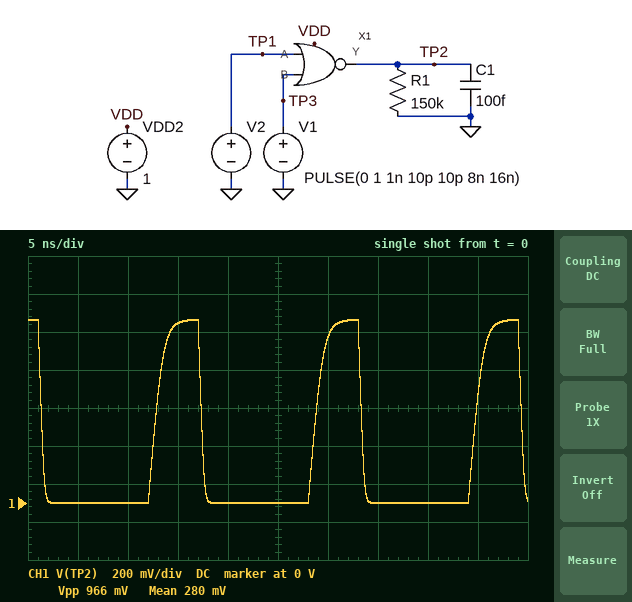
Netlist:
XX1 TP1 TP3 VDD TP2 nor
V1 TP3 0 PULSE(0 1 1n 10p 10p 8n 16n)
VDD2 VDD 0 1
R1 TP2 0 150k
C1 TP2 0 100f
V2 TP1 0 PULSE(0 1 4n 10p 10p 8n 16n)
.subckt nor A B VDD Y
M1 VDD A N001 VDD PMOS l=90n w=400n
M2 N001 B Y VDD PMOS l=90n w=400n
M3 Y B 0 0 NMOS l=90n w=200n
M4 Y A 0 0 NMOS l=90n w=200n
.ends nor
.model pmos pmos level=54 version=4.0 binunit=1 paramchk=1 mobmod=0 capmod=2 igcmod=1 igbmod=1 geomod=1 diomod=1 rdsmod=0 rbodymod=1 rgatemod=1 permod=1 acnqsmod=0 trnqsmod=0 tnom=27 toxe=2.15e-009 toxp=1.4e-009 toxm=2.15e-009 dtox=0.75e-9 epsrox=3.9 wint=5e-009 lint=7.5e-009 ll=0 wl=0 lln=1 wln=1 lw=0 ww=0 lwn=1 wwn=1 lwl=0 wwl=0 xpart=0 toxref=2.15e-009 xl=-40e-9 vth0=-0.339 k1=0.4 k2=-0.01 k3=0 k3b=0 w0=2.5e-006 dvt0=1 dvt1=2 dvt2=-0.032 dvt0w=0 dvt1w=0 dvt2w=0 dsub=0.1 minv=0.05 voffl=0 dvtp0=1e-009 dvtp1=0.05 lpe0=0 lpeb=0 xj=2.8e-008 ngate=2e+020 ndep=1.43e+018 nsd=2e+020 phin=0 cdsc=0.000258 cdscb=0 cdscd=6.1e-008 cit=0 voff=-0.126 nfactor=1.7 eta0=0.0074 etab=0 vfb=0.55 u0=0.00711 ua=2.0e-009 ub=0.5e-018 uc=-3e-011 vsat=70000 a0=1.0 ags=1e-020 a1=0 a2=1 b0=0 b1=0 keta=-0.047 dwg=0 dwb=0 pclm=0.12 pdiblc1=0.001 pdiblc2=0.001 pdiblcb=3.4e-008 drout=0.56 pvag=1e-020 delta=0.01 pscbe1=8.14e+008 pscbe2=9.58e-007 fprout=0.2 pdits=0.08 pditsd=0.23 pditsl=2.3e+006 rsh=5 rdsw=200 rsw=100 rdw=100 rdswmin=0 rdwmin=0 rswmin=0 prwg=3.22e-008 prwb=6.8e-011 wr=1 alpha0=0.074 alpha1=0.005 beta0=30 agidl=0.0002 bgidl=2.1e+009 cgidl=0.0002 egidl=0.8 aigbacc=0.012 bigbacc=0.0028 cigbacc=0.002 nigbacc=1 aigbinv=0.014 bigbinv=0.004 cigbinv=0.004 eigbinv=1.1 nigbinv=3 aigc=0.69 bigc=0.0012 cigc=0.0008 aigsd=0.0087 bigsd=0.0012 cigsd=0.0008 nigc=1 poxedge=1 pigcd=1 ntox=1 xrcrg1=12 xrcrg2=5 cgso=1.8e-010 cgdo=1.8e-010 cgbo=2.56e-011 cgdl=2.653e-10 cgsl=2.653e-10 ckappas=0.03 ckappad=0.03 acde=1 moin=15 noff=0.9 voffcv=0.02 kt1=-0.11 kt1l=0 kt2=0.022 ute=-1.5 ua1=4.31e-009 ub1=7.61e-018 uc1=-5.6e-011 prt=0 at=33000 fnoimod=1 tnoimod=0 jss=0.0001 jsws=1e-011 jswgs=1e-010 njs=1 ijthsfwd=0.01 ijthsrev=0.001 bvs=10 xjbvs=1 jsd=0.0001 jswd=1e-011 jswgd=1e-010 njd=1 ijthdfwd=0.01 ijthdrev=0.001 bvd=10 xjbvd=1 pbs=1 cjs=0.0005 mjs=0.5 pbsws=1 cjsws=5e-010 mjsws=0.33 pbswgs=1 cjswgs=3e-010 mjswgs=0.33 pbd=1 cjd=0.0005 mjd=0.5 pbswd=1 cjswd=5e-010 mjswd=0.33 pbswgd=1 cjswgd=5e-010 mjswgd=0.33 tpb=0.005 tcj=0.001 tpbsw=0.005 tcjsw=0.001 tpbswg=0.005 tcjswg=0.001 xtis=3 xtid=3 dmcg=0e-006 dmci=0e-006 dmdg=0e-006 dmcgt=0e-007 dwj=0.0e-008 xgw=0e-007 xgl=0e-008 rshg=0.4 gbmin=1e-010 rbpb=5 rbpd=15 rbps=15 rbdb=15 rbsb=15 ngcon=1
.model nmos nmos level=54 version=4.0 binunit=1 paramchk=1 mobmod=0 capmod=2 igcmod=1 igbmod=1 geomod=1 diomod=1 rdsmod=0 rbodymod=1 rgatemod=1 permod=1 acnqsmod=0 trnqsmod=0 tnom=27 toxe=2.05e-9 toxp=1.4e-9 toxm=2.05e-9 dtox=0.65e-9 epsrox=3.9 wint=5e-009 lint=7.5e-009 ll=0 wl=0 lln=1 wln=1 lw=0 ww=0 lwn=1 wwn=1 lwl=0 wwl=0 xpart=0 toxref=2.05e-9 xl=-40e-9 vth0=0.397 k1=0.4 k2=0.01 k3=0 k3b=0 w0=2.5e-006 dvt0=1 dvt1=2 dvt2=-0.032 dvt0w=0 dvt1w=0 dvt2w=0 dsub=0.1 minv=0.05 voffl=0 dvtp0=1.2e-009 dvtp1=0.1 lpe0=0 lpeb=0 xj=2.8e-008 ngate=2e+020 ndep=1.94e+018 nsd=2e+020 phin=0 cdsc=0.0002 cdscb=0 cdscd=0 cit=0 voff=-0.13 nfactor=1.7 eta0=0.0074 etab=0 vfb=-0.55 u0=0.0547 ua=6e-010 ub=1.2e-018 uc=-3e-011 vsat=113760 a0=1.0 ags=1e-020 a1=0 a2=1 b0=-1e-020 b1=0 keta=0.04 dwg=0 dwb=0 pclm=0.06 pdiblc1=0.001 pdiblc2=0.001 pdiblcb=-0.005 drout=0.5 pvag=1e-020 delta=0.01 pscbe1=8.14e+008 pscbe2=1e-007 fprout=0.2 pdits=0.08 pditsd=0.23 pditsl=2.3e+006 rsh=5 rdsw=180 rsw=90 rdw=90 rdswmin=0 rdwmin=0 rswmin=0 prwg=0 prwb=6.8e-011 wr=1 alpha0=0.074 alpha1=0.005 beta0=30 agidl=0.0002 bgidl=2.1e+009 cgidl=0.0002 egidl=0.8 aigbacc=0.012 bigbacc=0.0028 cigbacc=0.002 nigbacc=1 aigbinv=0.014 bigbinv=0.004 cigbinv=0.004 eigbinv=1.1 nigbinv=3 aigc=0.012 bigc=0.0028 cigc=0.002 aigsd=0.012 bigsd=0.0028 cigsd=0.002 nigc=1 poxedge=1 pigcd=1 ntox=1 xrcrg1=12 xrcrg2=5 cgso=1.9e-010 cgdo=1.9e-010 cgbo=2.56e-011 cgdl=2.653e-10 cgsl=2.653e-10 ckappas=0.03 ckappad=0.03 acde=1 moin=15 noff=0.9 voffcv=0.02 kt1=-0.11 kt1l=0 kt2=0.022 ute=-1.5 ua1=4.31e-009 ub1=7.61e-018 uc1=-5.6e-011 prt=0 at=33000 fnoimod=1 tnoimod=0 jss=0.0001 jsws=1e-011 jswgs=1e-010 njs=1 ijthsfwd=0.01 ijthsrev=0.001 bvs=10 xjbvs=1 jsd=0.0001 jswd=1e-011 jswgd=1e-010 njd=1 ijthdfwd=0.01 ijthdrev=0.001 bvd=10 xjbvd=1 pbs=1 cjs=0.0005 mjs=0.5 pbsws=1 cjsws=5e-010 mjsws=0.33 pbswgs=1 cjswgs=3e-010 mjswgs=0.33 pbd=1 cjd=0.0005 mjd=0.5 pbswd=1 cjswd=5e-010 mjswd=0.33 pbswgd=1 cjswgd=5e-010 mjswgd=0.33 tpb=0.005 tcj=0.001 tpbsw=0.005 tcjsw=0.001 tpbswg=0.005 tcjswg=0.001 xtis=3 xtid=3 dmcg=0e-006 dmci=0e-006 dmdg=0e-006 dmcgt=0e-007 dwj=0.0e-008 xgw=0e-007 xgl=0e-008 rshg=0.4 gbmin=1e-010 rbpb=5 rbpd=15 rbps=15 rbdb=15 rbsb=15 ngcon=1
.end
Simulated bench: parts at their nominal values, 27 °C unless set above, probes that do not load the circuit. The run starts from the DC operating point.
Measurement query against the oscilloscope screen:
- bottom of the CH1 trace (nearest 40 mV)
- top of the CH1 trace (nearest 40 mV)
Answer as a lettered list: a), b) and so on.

a) 0 V
b) 960 mV
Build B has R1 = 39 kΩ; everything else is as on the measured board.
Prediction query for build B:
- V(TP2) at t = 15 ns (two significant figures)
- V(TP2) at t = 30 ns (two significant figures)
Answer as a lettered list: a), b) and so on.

a) 850 mV
b) 780 mV
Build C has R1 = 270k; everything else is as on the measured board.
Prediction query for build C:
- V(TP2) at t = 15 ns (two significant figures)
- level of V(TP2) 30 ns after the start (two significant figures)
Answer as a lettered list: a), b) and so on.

a) 960 mV
b) 890 mV
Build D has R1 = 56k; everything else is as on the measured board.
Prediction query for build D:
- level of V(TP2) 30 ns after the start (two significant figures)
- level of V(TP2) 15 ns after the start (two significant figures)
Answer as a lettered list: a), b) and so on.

a) 820 mV
b) 890 mV
